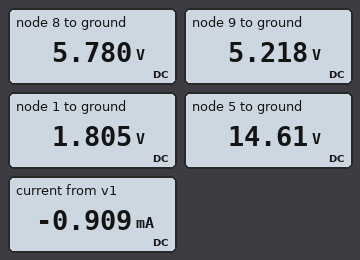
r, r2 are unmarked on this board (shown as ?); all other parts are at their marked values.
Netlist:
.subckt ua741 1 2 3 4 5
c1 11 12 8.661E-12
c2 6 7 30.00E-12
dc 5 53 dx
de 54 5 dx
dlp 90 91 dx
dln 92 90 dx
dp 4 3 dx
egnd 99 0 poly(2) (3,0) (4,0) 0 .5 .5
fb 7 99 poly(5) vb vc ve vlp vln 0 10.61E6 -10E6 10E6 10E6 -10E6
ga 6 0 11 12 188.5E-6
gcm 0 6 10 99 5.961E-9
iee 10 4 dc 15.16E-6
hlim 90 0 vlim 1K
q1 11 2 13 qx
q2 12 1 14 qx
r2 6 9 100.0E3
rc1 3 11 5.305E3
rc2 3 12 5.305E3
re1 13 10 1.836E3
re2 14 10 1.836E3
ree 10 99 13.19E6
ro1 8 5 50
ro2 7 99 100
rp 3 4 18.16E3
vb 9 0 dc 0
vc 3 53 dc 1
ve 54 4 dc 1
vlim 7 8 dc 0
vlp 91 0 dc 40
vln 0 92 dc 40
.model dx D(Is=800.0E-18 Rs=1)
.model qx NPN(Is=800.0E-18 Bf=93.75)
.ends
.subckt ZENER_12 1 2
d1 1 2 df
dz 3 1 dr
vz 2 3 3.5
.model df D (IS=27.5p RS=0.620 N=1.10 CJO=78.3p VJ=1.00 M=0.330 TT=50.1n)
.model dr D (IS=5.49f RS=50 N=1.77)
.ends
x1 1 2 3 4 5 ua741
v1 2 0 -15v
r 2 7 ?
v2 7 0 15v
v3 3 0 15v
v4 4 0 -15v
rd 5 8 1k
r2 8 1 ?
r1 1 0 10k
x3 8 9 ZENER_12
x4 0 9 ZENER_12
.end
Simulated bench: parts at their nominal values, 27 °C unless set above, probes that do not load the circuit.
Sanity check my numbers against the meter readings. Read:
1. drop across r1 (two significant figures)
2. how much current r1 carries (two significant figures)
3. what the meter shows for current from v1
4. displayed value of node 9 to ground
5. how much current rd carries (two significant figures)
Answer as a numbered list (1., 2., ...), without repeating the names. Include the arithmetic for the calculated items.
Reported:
1. 1.805 V = 1.8 V
2. (1.805 V) / 10 kΩ = 180 µA
3. -0.909 mA
4. 5.218 V
5. (14.61 V - 5.78 V) / 1 kΩ = 8.8 mA
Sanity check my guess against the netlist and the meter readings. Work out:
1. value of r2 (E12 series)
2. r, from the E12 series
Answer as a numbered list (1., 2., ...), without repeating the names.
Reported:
1. 22 kΩ
2. 33 kΩ
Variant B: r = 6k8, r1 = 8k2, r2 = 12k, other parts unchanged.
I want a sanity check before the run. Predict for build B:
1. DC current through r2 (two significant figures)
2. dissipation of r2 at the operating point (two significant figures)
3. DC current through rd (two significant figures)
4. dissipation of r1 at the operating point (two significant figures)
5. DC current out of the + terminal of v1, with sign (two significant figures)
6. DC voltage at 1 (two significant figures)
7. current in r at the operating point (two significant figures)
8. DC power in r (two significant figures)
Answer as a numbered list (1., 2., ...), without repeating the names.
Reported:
1. 290 µA
2. 980 µW
3. 8.8 mA
4. 670 µW
5. -4.4 mA
6. 2.3 V
7. 4.4 mA
8. 130 mW
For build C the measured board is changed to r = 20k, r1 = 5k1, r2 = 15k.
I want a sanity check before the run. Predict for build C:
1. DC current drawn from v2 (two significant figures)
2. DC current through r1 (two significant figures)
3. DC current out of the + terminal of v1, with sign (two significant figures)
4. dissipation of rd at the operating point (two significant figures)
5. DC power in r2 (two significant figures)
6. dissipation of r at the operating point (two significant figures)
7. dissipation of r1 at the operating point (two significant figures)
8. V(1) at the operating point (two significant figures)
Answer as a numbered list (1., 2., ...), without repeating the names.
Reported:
1. 1.5 mA
2. 290 µA
3. -1.5 mA
4. 78 mW
5. 1.2 mW
6. 45 mW
7. 420 µW
8. 1.5 V
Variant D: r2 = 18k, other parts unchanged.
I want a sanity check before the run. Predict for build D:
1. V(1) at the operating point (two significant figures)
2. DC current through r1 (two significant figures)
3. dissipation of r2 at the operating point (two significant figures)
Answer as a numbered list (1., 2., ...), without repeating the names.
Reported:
1. 2.1 V
2. 210 µA
3. 770 µW
